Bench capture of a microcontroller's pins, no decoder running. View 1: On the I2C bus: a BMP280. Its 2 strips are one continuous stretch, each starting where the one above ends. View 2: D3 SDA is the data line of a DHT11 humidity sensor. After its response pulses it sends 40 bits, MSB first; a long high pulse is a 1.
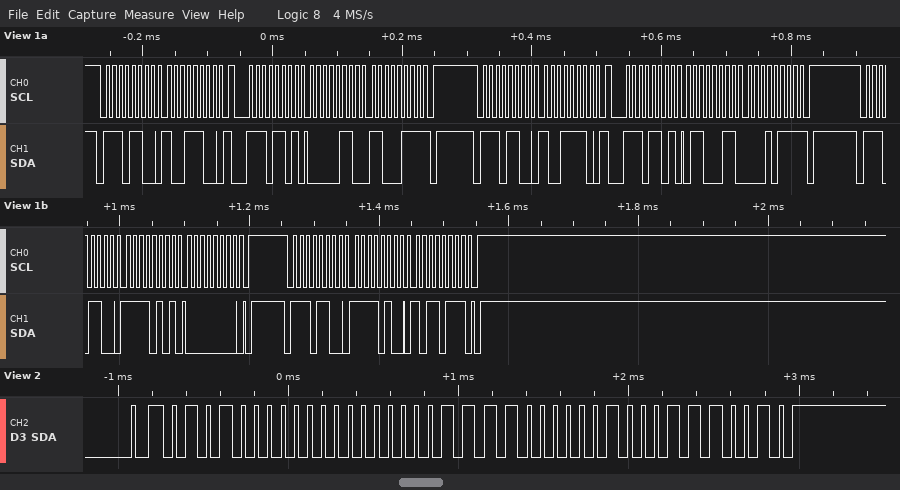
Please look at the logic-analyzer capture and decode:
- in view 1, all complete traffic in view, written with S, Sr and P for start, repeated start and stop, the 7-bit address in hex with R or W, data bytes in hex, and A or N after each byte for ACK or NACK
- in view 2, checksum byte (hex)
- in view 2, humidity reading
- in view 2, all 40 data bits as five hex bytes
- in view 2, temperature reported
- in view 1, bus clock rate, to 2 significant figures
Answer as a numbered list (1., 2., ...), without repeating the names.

1. S 76W A 9C A Sr 76R A 06 A C7 N P S 76W A 9E A Sr 76R A 63 A 17 N P S 76W A F5 A 00 A P S 76W A F4 A B7 A P
2. 0x72
3. 80 %
4. 50 00 1E 04 72
5. 30.4 °C
6. 100 kHz
